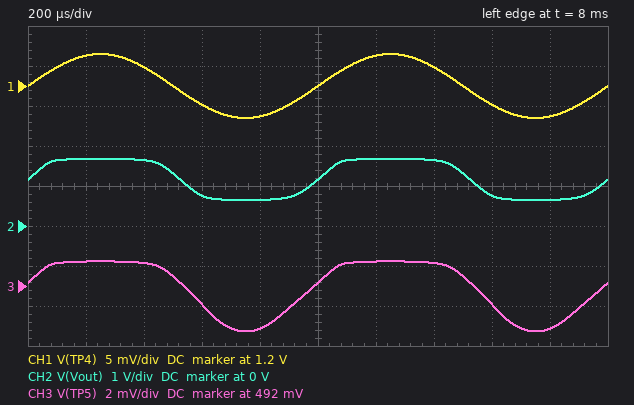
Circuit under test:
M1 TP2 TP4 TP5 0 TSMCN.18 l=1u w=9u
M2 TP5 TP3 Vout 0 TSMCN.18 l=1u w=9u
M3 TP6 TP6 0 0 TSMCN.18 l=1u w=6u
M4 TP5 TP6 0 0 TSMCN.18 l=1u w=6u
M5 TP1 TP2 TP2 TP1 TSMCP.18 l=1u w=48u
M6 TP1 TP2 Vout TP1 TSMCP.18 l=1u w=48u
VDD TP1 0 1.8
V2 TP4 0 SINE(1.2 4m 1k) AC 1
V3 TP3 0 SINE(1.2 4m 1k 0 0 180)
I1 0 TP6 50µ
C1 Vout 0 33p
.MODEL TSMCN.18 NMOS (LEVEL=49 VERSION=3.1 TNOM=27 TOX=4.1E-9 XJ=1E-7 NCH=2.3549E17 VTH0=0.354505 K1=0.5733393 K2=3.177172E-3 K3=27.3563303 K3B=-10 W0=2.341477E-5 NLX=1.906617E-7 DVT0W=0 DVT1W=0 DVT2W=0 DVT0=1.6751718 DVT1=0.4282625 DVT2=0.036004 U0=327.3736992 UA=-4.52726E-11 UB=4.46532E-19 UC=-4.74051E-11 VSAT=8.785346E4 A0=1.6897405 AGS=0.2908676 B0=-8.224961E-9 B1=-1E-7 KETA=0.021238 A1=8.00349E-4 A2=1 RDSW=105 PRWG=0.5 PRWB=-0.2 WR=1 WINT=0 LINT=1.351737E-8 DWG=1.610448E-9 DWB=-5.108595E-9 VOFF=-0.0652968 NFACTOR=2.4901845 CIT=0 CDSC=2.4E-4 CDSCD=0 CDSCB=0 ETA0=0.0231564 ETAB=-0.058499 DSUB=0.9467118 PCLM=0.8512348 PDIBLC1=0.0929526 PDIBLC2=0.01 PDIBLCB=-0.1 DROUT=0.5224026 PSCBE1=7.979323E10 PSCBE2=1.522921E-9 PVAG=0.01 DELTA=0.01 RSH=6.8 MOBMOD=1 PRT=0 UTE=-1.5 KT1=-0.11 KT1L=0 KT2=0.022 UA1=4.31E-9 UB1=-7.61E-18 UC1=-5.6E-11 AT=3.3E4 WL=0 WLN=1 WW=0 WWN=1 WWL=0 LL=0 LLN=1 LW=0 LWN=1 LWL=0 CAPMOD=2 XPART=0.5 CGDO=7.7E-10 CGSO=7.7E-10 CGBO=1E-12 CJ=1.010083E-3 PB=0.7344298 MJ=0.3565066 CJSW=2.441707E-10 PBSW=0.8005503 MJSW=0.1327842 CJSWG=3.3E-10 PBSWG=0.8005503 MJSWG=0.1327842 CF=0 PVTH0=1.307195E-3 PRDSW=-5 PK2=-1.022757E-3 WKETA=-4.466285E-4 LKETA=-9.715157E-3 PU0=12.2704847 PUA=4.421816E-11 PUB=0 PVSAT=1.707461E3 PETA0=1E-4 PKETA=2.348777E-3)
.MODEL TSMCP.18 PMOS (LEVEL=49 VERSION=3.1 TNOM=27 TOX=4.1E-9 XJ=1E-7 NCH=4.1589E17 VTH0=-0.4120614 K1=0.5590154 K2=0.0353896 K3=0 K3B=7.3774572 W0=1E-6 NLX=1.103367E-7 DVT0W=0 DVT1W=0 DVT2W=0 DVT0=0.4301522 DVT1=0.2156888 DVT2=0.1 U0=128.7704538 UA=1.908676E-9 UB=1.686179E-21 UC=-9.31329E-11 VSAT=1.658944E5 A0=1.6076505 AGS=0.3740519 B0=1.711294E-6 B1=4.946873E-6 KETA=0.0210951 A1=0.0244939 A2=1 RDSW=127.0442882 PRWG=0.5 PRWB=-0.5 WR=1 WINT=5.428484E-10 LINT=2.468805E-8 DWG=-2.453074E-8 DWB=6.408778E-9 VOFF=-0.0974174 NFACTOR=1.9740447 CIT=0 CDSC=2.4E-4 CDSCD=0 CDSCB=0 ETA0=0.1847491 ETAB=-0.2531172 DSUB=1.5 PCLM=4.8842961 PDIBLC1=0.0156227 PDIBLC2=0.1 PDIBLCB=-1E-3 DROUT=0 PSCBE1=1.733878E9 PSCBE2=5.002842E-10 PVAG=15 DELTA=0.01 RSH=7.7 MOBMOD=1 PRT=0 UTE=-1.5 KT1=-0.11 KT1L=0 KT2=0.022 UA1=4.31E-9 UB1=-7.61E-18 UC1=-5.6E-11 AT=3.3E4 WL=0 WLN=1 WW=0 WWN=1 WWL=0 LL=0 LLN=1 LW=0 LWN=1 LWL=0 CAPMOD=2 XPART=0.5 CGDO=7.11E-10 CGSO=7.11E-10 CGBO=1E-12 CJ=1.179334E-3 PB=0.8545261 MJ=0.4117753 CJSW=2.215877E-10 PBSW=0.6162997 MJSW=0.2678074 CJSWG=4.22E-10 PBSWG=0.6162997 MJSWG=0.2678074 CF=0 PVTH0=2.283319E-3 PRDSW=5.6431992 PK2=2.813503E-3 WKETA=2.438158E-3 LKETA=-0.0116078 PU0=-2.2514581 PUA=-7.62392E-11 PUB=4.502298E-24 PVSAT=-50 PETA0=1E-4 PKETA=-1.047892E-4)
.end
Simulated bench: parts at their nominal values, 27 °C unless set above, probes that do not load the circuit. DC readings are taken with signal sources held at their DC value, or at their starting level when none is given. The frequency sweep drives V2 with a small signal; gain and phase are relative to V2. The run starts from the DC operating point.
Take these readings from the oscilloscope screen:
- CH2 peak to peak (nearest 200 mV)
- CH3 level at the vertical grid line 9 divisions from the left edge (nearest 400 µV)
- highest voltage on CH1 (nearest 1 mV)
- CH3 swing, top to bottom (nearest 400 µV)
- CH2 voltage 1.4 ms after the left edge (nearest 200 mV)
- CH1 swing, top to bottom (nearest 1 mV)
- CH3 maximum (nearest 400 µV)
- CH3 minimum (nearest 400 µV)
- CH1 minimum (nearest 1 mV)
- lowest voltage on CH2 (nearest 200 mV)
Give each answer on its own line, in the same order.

1.0 V
490.0 mV
1.204 V
3.6 mV
1.6 V
8 mV
493.2 mV
489.6 mV
1.196 V
600 mV
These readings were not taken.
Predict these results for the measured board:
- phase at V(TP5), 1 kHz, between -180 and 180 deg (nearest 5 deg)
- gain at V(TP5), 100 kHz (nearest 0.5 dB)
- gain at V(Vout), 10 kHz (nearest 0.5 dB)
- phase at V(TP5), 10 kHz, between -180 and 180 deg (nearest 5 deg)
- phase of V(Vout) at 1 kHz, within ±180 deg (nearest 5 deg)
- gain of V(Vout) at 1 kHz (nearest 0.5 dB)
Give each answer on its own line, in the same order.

0 deg
-8.0 dB
40.0 dB
-15 deg
-5 deg
42.0 dB
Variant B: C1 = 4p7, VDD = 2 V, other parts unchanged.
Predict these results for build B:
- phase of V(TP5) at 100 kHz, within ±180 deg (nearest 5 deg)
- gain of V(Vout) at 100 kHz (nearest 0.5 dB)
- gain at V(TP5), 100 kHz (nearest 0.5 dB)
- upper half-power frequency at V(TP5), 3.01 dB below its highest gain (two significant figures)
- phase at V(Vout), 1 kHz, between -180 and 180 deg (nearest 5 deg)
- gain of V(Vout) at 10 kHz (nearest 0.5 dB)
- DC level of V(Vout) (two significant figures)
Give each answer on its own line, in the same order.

-15 deg
38.5 dB
-5.5 dB
160 kHz
0 deg
42.0 dB
1.4 V
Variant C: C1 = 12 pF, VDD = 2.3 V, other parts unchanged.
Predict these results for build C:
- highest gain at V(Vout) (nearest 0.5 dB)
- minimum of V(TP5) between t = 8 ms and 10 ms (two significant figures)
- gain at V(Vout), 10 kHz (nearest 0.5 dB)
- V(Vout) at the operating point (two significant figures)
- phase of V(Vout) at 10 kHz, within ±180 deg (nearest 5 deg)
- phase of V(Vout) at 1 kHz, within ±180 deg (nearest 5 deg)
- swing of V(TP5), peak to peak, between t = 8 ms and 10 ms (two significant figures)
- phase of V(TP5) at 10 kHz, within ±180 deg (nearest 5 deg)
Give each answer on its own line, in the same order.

42.5 dB
490 mV
42.0 dB
1.7 V
-15 deg
0 deg
3.1 mV
-5 deg
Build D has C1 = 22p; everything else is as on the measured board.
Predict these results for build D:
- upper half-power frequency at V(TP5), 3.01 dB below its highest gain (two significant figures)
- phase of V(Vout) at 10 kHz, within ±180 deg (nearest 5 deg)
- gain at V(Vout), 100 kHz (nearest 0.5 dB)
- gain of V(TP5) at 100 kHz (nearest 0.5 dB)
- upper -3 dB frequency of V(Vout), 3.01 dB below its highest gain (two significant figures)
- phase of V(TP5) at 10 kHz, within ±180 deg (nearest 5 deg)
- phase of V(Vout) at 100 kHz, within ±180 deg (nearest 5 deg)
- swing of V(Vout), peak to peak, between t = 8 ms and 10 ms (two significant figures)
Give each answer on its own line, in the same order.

36 kHz
-30 deg
27.5 dB
-7.5 dB
19 kHz
-10 deg
-80 deg
1.0 V
